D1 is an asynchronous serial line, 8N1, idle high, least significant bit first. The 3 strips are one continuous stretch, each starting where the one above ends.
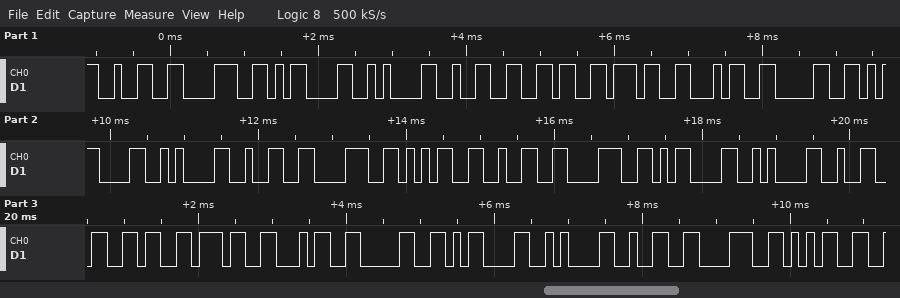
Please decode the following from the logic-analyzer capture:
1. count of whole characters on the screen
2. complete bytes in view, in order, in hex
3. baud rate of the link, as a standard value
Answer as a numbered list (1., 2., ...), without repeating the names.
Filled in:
1. 28
2. 32 38 0D 0A 32 36 37 34 30 0D 0A 32 38 35 32 38 0D 0A 32 36 37 34 30 0D 0A 32 38 35
3. 9600 baud
